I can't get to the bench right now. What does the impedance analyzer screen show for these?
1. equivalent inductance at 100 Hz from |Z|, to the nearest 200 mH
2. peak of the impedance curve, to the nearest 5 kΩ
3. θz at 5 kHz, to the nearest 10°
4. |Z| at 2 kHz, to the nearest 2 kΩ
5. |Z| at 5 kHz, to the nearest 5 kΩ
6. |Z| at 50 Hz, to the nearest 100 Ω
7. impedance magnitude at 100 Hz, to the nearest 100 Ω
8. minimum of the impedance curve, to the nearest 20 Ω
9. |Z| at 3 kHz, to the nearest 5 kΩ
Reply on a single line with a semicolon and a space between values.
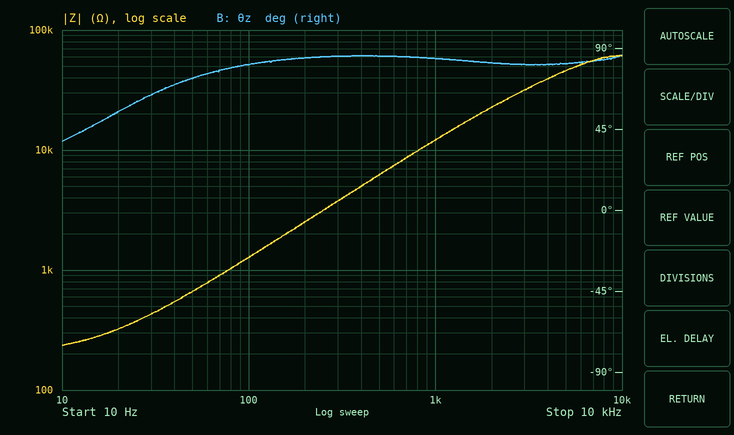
2.0 H; 60 kΩ; 80°; 22 kΩ; 45 kΩ; 700 Ω; 1.3 kΩ; 240 Ω; 30 kΩ
